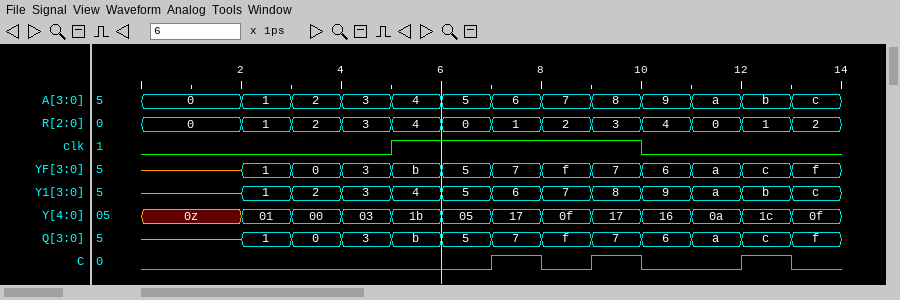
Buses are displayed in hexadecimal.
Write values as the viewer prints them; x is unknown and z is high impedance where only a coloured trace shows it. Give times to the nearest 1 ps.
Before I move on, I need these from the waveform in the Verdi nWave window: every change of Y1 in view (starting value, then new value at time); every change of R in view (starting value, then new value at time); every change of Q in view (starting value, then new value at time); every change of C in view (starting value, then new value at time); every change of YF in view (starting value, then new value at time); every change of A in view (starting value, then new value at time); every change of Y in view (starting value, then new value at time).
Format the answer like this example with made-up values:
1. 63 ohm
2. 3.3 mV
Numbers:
1. z, 1 at 2 ps, 2 at 3 ps, 3 at 4 ps, 4 at 5 ps, 5 at 6 ps, 6 at 7 ps, 7 at 8 ps, 8 at 9 ps, 9 at 10 ps, a at 11 ps, b at 12 ps, c at 13 ps
2. 0, 1 at 2 ps, 2 at 3 ps, 3 at 4 ps, 4 at 5 ps, 0 at 6 ps, 1 at 7 ps, 2 at 8 ps, 3 at 9 ps, 4 at 10 ps, 0 at 11 ps, 1 at 12 ps, 2 at 13 ps
3. z, 1 at 2 ps, 0 at 3 ps, 3 at 4 ps, b at 5 ps, 5 at 6 ps, 7 at 7 ps, f at 8 ps, 7 at 9 ps, 6 at 10 ps, a at 11 ps, c at 12 ps, f at 13 ps
4. 0, 1 at 7 ps, 0 at 8 ps, 1 at 9 ps, 0 at 10 ps, 1 at 12 ps, 0 at 13 ps
5. z, 1 at 2 ps, 0 at 3 ps, 3 at 4 ps, b at 5 ps, 5 at 6 ps, 7 at 7 ps, f at 8 ps, 7 at 9 ps, 6 at 10 ps, a at 11 ps, c at 12 ps, f at 13 ps
6. 0, 1 at 2 ps, 2 at 3 ps, 3 at 4 ps, 4 at 5 ps, 5 at 6 ps, 6 at 7 ps, 7 at 8 ps, 8 at 9 ps, 9 at 10 ps, a at 11 ps, b at 12 ps, c at 13 ps
7. 0z, 01 at 2 ps, 00 at 3 ps, 03 at 4 ps, 1b at 5 ps, 05 at 6 ps, 17 at 7 ps, 0f at 8 ps, 17 at 9 ps, 16 at 10 ps, 0a at 11 ps, 1c at 12 ps, 0f at 13 ps
